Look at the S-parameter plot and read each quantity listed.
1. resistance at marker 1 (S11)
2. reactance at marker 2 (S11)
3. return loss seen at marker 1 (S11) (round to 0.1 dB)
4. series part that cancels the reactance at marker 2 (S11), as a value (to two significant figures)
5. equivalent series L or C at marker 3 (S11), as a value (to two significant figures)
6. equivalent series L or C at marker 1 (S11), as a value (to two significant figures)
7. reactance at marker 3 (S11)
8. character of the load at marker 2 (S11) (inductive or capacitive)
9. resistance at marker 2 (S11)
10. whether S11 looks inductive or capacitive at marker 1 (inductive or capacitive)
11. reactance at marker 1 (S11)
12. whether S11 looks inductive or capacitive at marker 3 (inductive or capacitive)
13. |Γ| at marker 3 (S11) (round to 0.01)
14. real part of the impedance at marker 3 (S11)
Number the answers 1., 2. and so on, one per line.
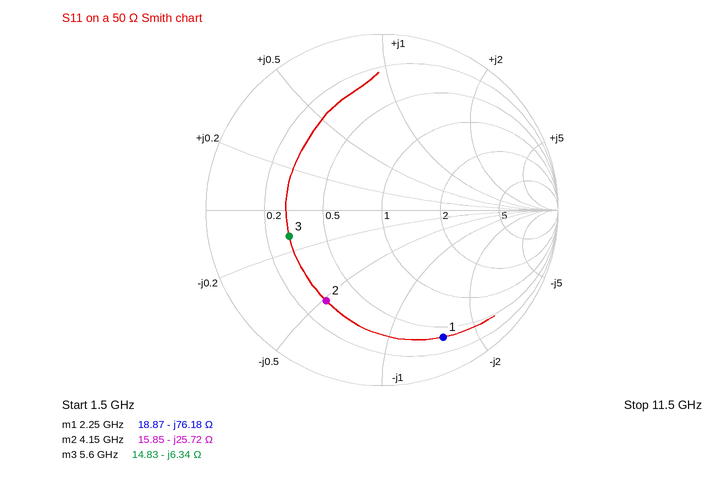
1. 18.87 Ω
2. -25.72 Ω
3. 1.9 dB
4. 990 pH
5. 4.5 pF
6. 930 fF
7. -6.34 Ω
8. capacitive
9. 15.85 Ω
10. capacitive
11. -76.18 Ω
12. capacitive
13. 0.55
14. 14.83 Ω
